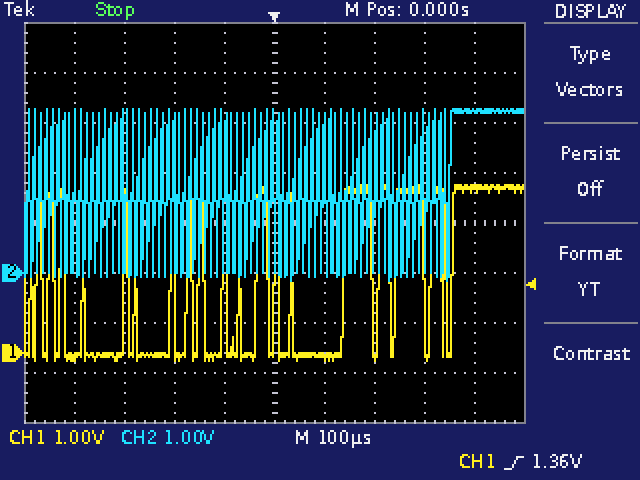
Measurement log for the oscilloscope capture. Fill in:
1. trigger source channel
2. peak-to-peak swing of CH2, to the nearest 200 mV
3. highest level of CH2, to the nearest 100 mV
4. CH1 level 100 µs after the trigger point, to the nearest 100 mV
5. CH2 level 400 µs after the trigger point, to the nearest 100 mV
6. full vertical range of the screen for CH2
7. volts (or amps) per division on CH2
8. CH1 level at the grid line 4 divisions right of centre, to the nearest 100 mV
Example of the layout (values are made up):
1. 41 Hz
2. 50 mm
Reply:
1. CH1
2. 3.4 V
3. 3.3 V
4. -100 mV
5. 3.2 V
6. 8 V
7. 1 V
8. 3.3 V
